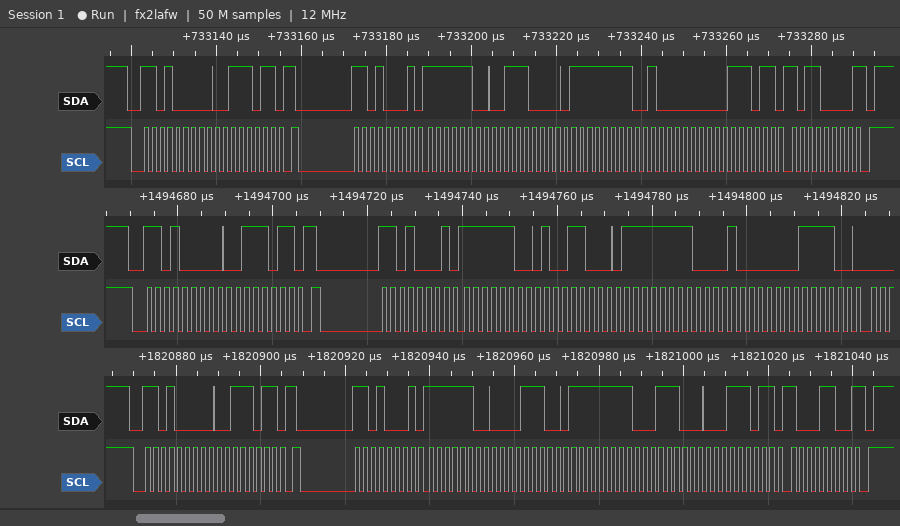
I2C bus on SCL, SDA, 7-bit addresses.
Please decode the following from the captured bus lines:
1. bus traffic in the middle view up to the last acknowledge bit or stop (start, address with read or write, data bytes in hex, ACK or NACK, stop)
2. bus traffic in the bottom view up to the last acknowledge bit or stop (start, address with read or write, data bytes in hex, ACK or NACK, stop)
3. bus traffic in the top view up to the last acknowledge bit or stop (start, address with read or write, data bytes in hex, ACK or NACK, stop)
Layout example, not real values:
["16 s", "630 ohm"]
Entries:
["start, address 68 write ACK, 3B ACK, repeated start, address 68 read ACK, FC ACK, 98 ACK, FF ACK, 10 ACK, 3C ACK", "start, address 68 write ACK, 3B ACK, repeated start, address 68 read ACK, FC ACK, 1C ACK, FF ACK, 38 ACK, 3B ACK, 8C NACK, stop", "start, address 68 write ACK, 3B ACK, repeated start, address 68 read ACK, FC ACK, 70 ACK, FF ACK, 40 ACK, 3B ACK, B0 NACK, stop"]
